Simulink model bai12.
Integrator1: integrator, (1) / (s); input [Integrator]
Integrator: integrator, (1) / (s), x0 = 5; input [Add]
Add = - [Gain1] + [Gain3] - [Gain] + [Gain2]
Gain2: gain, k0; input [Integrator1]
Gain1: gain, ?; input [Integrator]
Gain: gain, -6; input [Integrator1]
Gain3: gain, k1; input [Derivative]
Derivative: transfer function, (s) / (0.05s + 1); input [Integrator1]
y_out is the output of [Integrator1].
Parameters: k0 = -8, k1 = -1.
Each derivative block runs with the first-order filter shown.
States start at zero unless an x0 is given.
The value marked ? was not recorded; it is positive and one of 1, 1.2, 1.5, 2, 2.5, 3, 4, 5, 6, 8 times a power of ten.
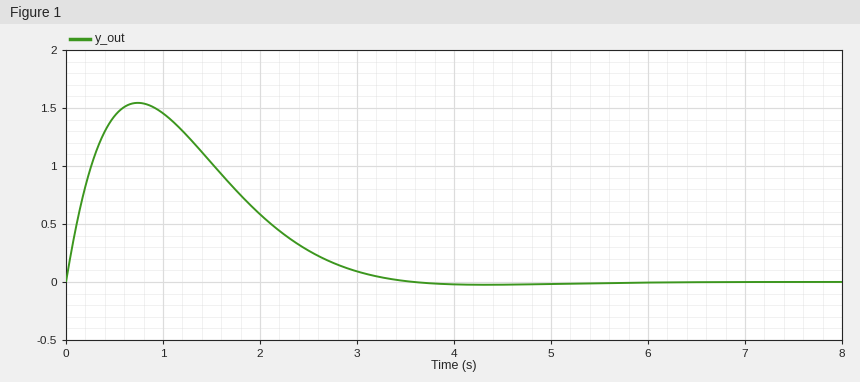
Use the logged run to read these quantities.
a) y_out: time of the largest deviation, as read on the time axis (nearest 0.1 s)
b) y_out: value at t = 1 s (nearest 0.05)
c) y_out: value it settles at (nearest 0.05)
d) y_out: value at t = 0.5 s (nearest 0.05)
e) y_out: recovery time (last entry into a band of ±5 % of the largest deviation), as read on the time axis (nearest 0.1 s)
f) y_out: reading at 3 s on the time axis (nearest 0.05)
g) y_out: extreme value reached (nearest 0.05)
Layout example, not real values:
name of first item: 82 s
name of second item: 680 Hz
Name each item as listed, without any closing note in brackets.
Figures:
y_out: time of the largest deviation, as read on the time axis: 0.7 s
y_out: value at t = 1 s: 1.45
y_out: value it settles at: 0.00
y_out: value at t = 0.5 s: 1.45
y_out: recovery time (last entry into a band of ±5 % of the largest deviation), as read on the time axis: 3.1 s
y_out: reading at 3 s on the time axis: 0.10
y_out: extreme value reached: 1.55
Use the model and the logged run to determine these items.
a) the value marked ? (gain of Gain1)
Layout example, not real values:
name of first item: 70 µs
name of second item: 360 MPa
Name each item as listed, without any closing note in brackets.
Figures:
the value marked ?: 1.2
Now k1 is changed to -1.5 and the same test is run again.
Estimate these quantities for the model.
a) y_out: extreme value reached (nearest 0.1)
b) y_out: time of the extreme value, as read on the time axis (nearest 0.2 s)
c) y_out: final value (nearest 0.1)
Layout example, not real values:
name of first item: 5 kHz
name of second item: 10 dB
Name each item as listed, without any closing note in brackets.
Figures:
y_out: extreme value reached: 1.4
y_out: time of the extreme value, as read on the time axis: 0.6 s
y_out: final value: 0.0
